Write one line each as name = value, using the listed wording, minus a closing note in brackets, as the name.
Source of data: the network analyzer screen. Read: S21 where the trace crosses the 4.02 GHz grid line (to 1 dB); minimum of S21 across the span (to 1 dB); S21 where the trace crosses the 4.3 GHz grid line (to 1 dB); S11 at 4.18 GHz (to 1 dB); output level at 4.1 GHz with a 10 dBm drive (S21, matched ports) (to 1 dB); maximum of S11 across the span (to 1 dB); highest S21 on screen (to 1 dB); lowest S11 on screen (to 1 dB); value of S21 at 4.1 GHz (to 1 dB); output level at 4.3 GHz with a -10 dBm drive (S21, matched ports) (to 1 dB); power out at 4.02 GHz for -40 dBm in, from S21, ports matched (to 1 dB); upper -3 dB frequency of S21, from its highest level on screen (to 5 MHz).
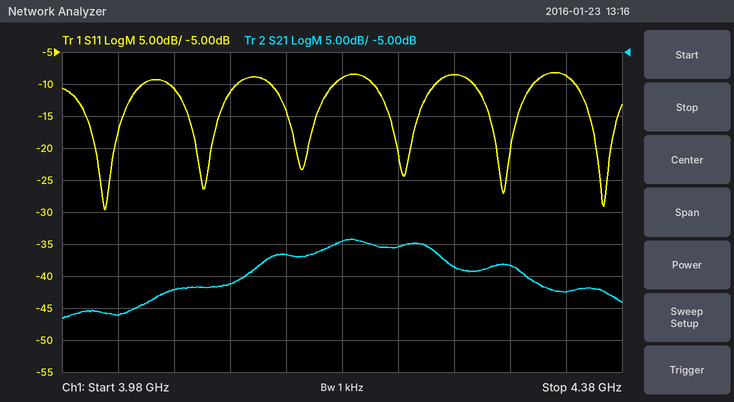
S21 where the trace crosses the 4.02 GHz grid line = -46 dB
minimum of S21 across the span = -47 dB
S21 where the trace crosses the 4.3 GHz grid line = -38 dB
S11 at 4.18 GHz = -9 dB
output level at 4.1 GHz with a 10 dBm drive (S21, matched ports) = -31 dBm
maximum of S11 across the span = -8 dB
highest S21 on screen = -34 dB
lowest S11 on screen = -30 dB
value of S21 at 4.1 GHz = -41 dB
output level at 4.3 GHz with a -10 dBm drive (S21, matched ports) = -48 dBm
power out at 4.02 GHz for -40 dBm in, from S21, ports matched = -86 dBm
upper -3 dB frequency of S21, from its highest level on screen = 4.250 GHz
